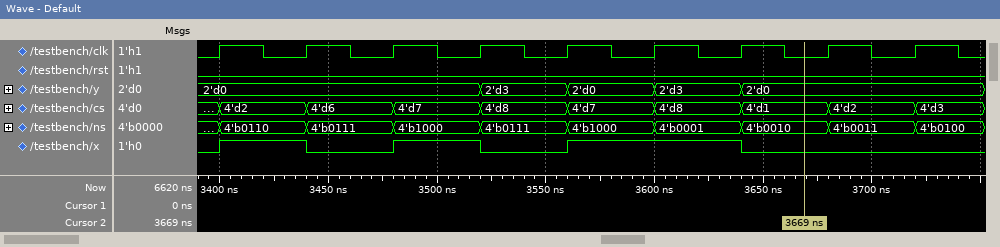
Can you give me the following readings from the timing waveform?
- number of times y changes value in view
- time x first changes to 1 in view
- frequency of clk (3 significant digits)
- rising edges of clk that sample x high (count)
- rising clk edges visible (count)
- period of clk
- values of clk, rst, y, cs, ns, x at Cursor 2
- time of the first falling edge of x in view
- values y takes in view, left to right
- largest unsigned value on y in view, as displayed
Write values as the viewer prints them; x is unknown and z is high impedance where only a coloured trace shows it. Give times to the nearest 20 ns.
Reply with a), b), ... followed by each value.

a) 4
b) 3400 ns
c) 25.0 MHz
d) 4
e) 9
f) 40 ns
g) clk=0, rst=0, y=2'd0, cs=4'd1, ns=4'b0010, x=0
h) 3440 ns
i) 2'd0, 2'd3, 2'd0, 2'd3, 2'd0
j) 2'd3
